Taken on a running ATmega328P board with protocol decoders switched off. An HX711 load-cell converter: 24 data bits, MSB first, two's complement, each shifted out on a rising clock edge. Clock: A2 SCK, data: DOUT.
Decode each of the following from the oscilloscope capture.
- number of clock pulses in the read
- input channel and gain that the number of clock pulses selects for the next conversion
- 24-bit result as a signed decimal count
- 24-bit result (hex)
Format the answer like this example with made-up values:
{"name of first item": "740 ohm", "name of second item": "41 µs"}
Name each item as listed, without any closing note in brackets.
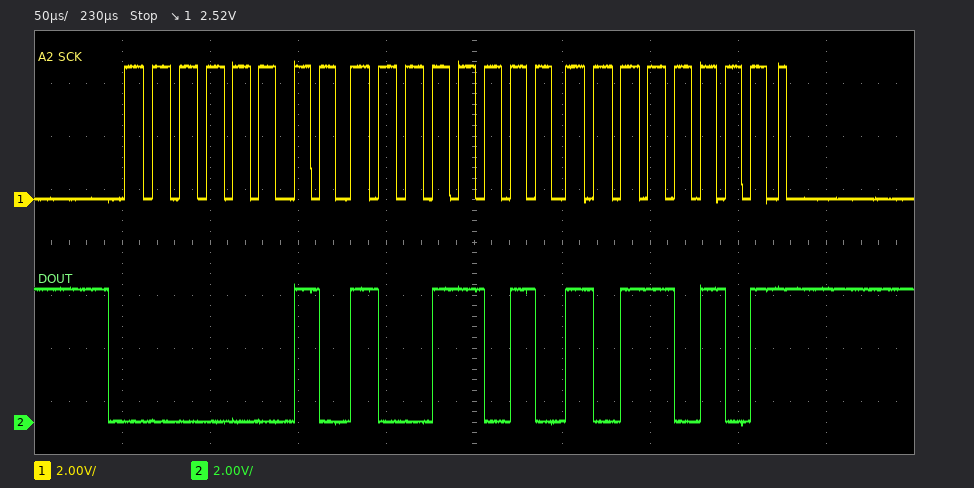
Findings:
{"number of clock pulses in the read": "25", "input channel and gain that the number of clock pulses selects for the next conversion": "channel A, gain 128", "24-bit result as a signed decimal count": "170677", "24-bit result": "0x029AB5"}
